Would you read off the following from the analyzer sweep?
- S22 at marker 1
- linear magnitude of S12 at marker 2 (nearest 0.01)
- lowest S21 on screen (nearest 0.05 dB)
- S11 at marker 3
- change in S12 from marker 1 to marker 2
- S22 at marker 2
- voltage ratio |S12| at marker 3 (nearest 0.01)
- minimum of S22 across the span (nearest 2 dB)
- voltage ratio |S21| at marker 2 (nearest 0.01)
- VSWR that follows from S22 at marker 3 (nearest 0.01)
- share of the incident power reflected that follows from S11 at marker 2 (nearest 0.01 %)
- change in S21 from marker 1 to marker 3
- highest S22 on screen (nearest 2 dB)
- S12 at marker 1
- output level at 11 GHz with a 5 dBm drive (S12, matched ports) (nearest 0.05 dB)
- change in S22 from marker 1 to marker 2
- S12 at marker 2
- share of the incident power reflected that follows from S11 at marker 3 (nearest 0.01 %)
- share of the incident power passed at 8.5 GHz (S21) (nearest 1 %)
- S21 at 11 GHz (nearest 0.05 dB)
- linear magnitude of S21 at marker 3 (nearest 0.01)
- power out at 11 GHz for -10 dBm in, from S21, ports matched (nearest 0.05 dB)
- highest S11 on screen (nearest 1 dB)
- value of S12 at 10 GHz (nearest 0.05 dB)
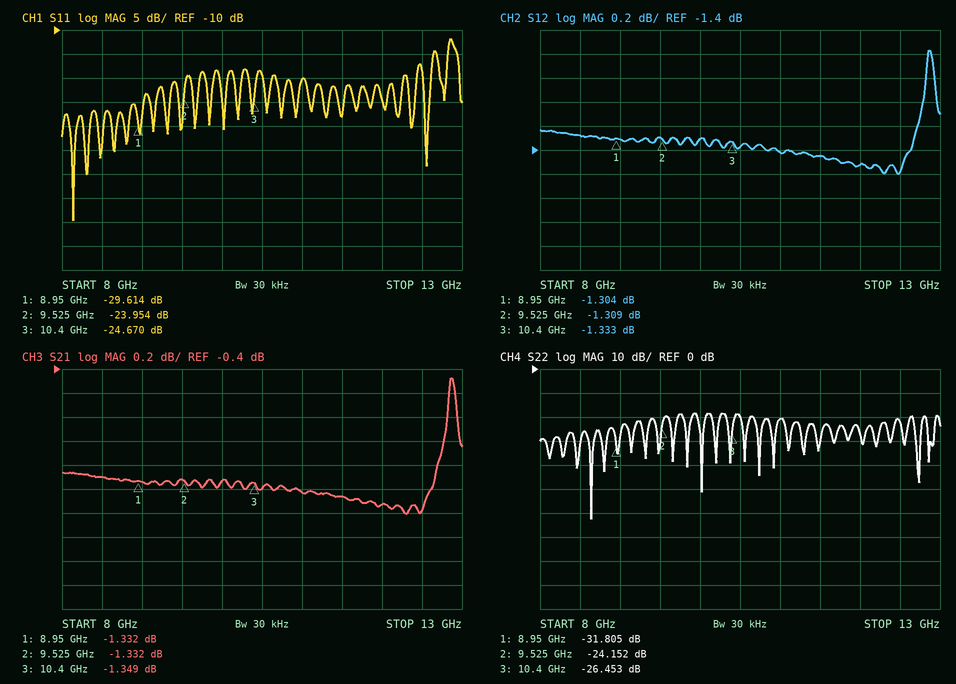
-31.805 dB
0.86
-1.60 dB
-24.670 dB
-0.005 dB
-24.152 dB
0.86
-62 dB
0.86
1.10
0.40 %
-0.017 dB
-18 dB
-1.304 dB
3.60 dBm
7.653 dB
-1.309 dB
0.34 %
74 %
-1.45 dB
0.86
-11.45 dBm
-12 dB
-1.30 dB
